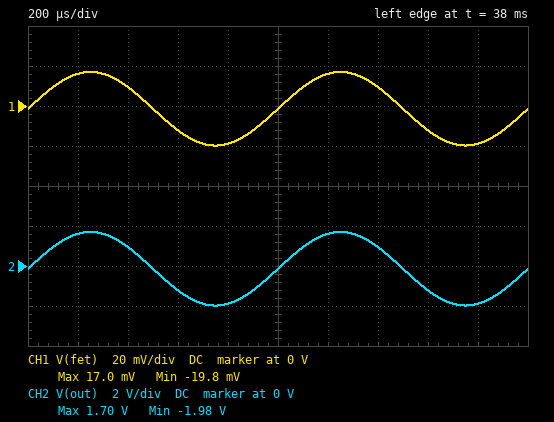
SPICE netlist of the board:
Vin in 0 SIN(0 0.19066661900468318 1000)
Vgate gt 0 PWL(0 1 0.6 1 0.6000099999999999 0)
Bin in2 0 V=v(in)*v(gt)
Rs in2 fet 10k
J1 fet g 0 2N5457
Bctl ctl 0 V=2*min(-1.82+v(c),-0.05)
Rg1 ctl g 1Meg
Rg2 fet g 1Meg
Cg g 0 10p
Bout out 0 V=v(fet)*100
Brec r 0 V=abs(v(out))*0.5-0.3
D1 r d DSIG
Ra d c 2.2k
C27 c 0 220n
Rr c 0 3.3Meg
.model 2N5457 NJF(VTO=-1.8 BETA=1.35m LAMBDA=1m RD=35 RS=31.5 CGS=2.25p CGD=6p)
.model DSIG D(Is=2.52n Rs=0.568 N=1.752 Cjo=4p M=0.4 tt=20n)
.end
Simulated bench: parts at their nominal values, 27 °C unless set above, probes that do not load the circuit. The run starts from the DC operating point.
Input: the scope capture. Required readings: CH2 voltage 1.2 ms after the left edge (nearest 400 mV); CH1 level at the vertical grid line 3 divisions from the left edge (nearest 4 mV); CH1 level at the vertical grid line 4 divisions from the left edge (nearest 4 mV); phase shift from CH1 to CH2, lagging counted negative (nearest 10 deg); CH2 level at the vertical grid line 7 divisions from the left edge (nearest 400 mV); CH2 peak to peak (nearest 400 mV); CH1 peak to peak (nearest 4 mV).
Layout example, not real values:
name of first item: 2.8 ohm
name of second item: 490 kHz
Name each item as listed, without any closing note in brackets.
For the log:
CH2 voltage 1.2 ms after the left edge: 1.6 V
CH1 level at the vertical grid line 3 divisions from the left edge: -12 mV
CH1 level at the vertical grid line 4 divisions from the left edge: -20 mV
phase shift from CH1 to CH2, lagging counted negative: 0 deg
CH2 level at the vertical grid line 7 divisions from the left edge: 800 mV
CH2 peak to peak: 3.6 V
CH1 peak to peak: 36 mV
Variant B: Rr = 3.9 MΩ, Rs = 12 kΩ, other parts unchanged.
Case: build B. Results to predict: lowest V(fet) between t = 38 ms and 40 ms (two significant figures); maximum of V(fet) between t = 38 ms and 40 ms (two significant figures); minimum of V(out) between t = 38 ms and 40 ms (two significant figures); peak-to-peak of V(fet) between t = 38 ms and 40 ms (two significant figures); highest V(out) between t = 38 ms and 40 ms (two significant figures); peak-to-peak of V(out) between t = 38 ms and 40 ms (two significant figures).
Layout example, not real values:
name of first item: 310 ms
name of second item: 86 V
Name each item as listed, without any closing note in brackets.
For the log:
lowest V(fet) between t = 38 ms and 40 ms: -19 mV
maximum of V(fet) between t = 38 ms and 40 ms: 16 mV
minimum of V(out) between t = 38 ms and 40 ms: -1.9 V
peak-to-peak of V(fet) between t = 38 ms and 40 ms: 34 mV
highest V(out) between t = 38 ms and 40 ms: 1.6 V
peak-to-peak of V(out) between t = 38 ms and 40 ms: 3.4 V
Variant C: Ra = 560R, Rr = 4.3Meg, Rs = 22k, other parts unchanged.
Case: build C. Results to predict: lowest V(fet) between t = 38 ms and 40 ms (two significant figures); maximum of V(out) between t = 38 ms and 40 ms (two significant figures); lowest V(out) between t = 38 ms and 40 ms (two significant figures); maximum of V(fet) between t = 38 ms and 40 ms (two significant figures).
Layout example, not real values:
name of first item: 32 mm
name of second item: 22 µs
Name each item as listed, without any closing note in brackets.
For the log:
lowest V(fet) between t = 38 ms and 40 ms: -16 mV
maximum of V(out) between t = 38 ms and 40 ms: 1.1 V
lowest V(out) between t = 38 ms and 40 ms: -1.6 V
maximum of V(fet) between t = 38 ms and 40 ms: 11 mV
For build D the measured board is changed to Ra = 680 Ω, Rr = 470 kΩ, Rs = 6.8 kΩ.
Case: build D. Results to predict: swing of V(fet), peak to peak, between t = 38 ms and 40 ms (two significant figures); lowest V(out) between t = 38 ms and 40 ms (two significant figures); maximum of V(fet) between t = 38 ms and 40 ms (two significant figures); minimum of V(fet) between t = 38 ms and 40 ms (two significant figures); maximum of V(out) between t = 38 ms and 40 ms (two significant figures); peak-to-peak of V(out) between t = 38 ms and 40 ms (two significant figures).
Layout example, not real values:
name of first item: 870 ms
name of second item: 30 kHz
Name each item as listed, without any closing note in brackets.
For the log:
swing of V(fet), peak to peak, between t = 38 ms and 40 ms: 44 mV
lowest V(out) between t = 38 ms and 40 ms: -2.3 V
maximum of V(fet) between t = 38 ms and 40 ms: 21 mV
minimum of V(fet) between t = 38 ms and 40 ms: -23 mV
maximum of V(out) between t = 38 ms and 40 ms: 2.1 V
peak-to-peak of V(out) between t = 38 ms and 40 ms: 4.4 V
